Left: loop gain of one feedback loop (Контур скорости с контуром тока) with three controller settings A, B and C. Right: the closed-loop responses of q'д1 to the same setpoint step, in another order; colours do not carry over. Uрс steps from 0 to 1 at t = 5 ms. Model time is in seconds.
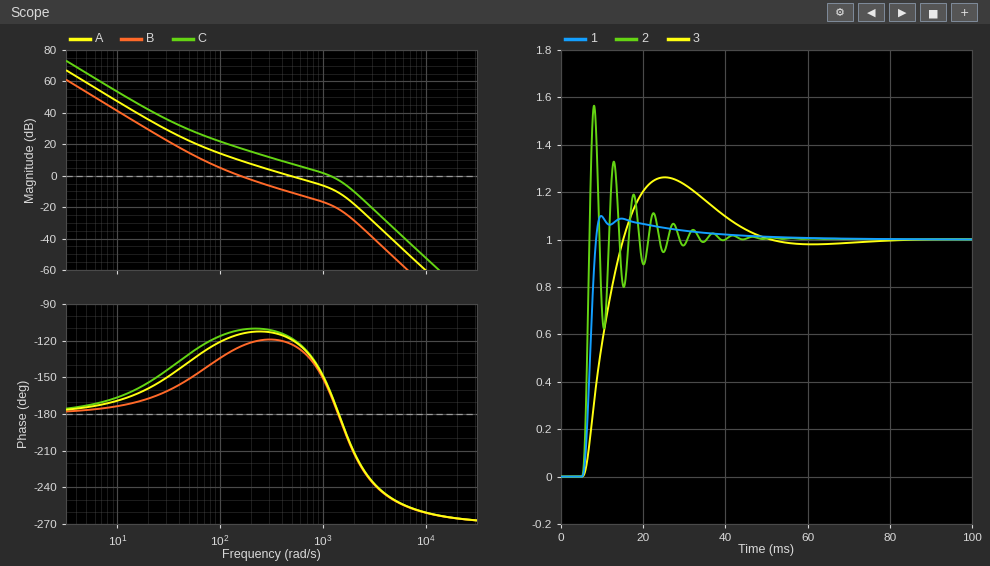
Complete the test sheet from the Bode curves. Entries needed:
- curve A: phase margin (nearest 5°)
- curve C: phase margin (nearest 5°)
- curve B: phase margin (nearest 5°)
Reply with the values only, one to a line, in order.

60°
20°
55°
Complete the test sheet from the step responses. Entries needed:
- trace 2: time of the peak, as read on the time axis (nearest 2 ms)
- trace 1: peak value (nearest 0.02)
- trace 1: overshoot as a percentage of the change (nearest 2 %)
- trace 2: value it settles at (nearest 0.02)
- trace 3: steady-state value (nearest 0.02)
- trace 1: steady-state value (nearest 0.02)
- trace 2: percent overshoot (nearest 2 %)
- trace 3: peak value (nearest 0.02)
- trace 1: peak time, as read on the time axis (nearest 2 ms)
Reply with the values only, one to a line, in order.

8 ms
1.10
10 %
1.00
1.00
1.00
56 %
1.26
10 ms
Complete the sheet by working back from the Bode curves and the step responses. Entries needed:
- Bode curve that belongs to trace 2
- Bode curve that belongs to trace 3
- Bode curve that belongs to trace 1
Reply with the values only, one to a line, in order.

C
B
A
